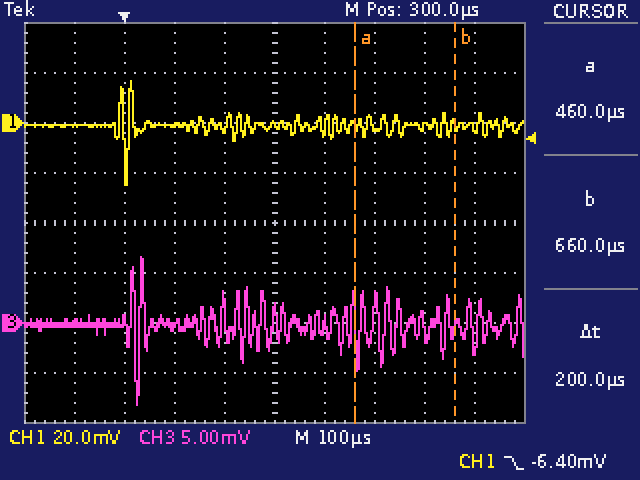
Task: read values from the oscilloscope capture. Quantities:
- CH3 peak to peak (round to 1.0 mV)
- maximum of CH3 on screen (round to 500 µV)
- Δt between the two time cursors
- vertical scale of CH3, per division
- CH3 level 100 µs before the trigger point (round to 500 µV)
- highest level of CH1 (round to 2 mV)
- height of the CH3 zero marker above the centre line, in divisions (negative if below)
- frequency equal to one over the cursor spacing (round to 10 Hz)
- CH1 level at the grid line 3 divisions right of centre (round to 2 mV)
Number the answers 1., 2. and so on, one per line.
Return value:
1. 15.0 mV
2. 6.5 mV
3. 200 µs
4. 5 mV
5. 0.0 mV
6. 16 mV
7. -2.0 div
8. 5.00 kHz
9. -2 mV
